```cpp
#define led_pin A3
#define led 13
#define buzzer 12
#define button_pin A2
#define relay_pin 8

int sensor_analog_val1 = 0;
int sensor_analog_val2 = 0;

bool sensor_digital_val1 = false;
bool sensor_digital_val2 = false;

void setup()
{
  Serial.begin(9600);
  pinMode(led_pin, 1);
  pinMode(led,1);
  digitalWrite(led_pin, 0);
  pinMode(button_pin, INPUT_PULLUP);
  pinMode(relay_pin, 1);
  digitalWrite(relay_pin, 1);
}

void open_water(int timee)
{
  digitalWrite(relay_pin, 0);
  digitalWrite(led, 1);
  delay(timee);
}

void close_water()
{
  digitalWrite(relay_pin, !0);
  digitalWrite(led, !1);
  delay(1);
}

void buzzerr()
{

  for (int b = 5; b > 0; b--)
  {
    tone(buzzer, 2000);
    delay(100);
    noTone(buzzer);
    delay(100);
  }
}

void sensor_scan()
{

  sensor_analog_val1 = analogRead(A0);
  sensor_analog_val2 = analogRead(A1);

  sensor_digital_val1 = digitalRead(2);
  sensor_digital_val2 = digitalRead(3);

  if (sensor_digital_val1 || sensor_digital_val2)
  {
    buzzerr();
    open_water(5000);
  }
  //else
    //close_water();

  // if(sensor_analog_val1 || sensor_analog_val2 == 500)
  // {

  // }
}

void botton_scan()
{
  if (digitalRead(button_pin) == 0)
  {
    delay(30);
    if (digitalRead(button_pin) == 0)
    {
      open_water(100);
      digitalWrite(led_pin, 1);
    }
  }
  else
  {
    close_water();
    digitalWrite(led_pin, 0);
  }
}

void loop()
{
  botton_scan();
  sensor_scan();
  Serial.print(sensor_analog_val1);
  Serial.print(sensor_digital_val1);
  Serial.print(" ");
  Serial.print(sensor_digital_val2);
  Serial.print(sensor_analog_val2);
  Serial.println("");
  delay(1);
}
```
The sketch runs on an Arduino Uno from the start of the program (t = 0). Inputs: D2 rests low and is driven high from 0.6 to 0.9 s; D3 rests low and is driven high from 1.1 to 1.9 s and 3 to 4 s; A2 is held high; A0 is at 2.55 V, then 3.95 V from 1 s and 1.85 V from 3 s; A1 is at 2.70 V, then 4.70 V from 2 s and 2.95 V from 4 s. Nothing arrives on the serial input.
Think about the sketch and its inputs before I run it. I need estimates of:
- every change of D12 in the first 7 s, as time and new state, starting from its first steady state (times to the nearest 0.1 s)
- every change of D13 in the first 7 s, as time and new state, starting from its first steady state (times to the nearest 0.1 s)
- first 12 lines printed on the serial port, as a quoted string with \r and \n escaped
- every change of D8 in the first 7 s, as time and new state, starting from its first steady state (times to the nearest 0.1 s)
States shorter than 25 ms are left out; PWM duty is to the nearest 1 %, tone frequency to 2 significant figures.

0.6 s tone 2000 Hz; 0.7 s low; 0.8 s tone 2000 Hz; 0.9 s low; 1 s tone 2000 Hz; 1.1 s low; 1.2 s tone 2000 Hz; 1.3 s low; 1.4 s tone 2000 Hz; 1.5 s low
0 s low; 1.6 s high; 6.6 s low
"5220 0552\r\n5220 0552\r\n5220 0552\r\n5220 0552\r\n5220 0552\r\n5220 0552\r\n5220 0552\r\n5220 0552\r\n5220 0552\r\n5220 0552\r\n5220 0552\r\n5220 0552\r\n"
0 s high; 1.6 s low; 6.6 s high
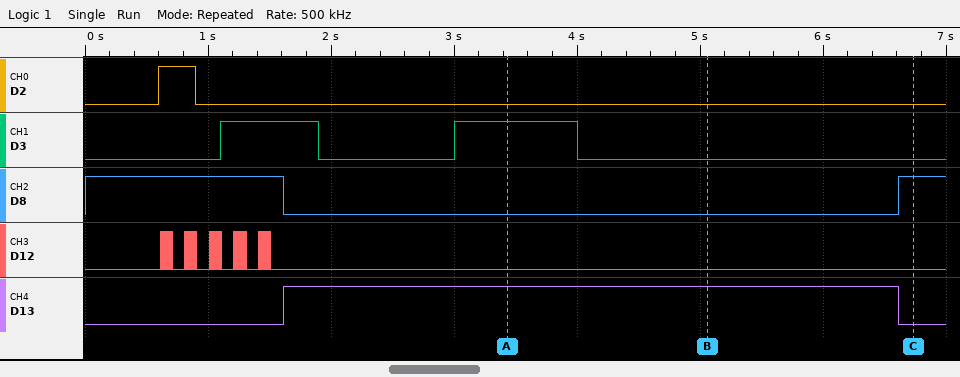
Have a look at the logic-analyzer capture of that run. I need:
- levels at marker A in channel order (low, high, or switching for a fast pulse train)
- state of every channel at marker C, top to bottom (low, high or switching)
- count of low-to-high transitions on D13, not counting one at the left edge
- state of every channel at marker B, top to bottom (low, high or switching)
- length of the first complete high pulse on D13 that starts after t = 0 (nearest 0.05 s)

D2 low, D3 high, D8 low, D12 low, D13 high
D2 low, D3 low, D8 high, D12 low, D13 low
1
D2 low, D3 low, D8 low, D12 low, D13 high
5.00 s
